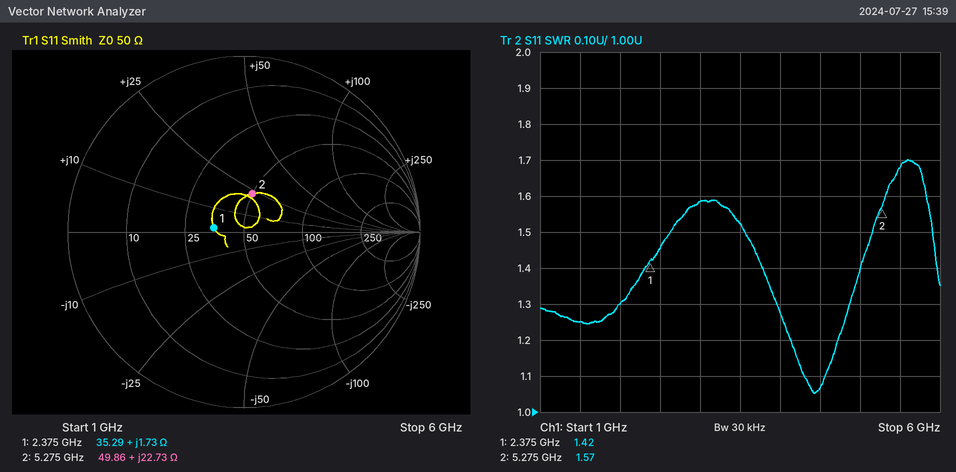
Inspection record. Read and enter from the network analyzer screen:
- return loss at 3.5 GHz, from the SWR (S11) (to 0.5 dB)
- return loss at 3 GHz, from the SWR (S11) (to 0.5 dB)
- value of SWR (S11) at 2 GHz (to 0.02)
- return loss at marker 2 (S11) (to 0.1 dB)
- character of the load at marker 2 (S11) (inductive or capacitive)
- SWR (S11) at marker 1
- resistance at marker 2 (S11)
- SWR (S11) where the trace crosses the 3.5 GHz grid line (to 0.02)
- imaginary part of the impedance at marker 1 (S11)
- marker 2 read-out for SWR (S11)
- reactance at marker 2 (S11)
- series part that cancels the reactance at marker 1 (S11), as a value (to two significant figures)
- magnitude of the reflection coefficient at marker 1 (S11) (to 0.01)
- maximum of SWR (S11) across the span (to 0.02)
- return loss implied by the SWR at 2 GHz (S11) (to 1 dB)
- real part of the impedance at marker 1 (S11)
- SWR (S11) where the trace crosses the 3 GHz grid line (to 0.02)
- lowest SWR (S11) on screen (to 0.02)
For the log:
13.5 dB
13.0 dB
1.30
13.1 dB
inductive
1.42
49.86 Ω
1.52
+1.73 Ω
1.57
+22.73 Ω
39 pF
0.17
1.70
18 dB
35.29 Ω
1.58
1.06
